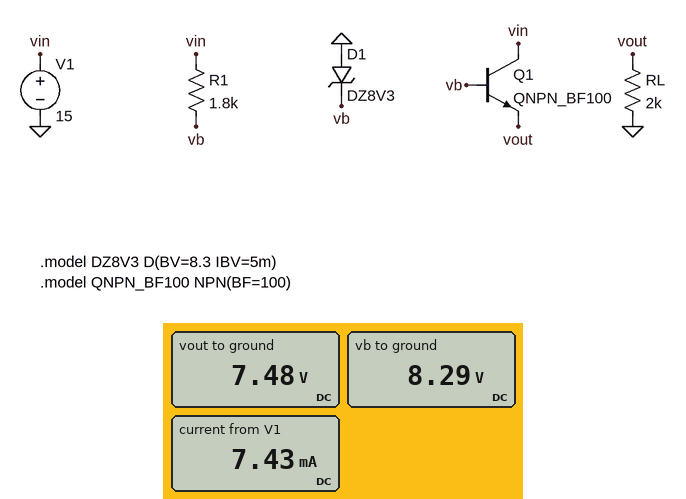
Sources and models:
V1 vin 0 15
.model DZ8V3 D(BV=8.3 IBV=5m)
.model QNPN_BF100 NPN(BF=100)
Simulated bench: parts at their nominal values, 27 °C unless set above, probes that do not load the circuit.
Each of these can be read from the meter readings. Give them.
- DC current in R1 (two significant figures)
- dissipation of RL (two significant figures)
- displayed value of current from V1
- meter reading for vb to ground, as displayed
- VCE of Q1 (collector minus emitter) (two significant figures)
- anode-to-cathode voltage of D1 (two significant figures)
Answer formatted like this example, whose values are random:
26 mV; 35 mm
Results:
3.7 mA; 28 mW; 7.43 mA; 8.29 V; 7.5 V; -8.3 V
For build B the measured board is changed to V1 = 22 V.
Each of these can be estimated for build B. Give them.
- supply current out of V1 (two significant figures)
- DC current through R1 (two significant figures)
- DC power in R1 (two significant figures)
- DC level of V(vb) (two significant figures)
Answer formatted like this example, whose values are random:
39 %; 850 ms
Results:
11 mA; 7.6 mA; 100 mW; 8.3 V
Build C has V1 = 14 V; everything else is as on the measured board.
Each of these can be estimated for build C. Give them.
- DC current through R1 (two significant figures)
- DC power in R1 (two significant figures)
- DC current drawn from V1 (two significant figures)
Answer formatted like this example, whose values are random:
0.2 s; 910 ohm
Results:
3.2 mA; 18 mW; 6.9 mA
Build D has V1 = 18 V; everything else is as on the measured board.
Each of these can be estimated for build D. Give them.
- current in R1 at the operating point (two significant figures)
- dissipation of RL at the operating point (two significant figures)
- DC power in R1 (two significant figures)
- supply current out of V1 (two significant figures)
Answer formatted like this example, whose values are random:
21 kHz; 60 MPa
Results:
5.4 mA; 28 mW; 52 mW; 9.1 mA
